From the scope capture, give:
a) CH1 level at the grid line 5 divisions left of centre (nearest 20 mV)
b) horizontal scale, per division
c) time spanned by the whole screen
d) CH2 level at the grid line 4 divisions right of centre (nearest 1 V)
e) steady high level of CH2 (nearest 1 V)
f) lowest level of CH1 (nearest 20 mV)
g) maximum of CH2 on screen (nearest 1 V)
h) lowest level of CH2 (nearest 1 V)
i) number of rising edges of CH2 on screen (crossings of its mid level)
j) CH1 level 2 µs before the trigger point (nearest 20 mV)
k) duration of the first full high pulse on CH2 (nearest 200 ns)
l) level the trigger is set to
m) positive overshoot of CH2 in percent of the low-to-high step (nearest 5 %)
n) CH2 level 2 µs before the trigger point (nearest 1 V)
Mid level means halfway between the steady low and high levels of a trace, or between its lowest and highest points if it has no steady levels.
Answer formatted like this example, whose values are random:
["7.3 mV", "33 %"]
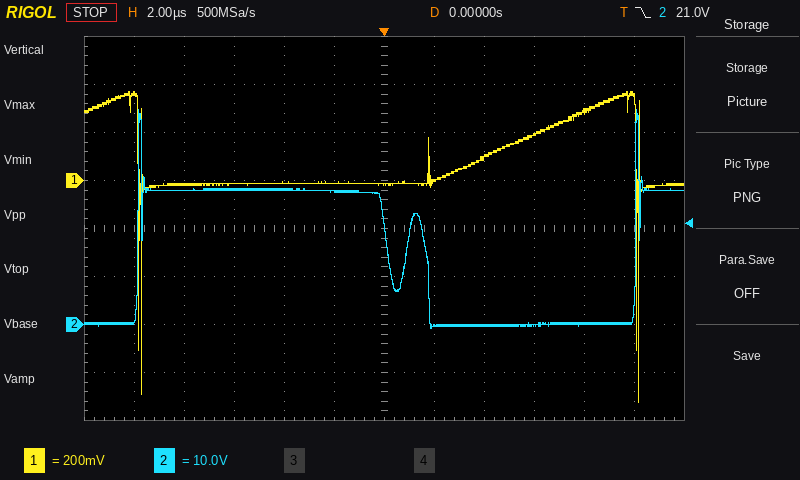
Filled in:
["360 mV", "2 µs", "24 µs", "0 V", "28 V", "-920 mV", "45 V", "-1 V", "3", "-20 mV", "10.0 µs", "21.0 V", "60 %", "28 V"]
